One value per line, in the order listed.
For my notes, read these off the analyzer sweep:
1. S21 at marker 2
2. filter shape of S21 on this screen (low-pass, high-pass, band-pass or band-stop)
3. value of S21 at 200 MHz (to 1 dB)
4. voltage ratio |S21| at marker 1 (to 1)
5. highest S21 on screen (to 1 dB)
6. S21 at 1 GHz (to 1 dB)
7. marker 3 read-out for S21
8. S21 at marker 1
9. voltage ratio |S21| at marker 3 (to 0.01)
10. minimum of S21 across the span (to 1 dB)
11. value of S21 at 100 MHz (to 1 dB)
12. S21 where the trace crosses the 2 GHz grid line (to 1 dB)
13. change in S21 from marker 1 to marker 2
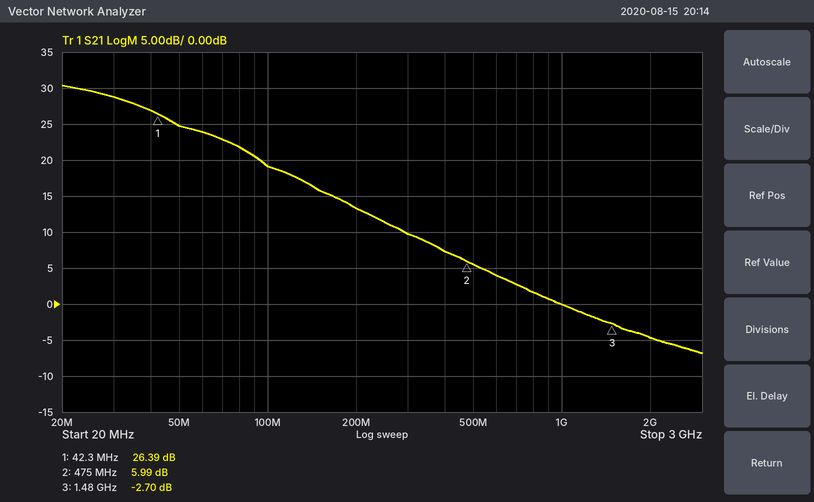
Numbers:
5.99 dB
low-pass
13 dB
21
30 dB
0 dB
-2.70 dB
26.39 dB
0.73
-7 dB
19 dB
-5 dB
-20.40 dB
